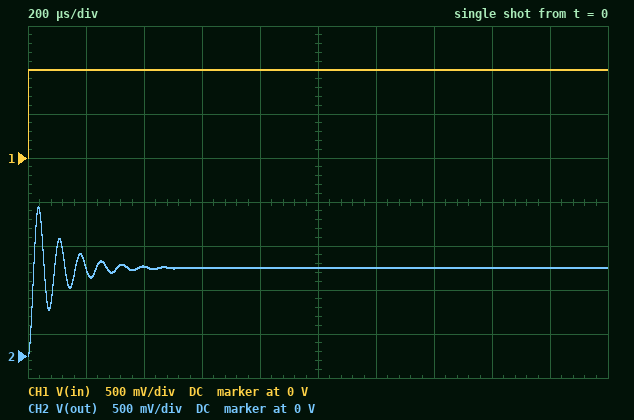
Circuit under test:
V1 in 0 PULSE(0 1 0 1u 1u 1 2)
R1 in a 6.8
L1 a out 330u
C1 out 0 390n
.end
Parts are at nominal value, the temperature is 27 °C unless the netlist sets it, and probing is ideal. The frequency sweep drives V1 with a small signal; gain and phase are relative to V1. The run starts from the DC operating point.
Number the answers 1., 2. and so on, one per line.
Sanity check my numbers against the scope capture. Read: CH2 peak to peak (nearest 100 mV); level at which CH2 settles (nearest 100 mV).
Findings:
1. 1.7 V
2. 1.0 V
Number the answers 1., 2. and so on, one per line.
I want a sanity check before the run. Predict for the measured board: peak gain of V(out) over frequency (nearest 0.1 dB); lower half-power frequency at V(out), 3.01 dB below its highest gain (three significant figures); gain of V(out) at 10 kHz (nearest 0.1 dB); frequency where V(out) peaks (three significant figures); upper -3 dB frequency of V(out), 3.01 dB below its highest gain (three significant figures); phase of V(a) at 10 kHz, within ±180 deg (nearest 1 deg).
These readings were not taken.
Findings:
1. 12.7 dB
2. 12.1 kHz
3. 5.7 dB
4. 13.8 kHz
5. 15.4 kHz
6. -19 deg
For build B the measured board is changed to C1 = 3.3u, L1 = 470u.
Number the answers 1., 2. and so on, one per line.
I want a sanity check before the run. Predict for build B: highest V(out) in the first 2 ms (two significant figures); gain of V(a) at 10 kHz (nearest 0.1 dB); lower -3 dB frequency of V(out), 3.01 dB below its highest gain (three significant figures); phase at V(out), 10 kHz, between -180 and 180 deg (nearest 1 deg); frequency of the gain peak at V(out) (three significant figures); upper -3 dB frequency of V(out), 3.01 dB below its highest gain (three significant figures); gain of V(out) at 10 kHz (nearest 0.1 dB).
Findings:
1. 1.4 V
2. -0.3 dB
3. 2.18 kHz
4. -165 deg
5. 3.70 kHz
6. 4.75 kHz
7. -14.5 dB
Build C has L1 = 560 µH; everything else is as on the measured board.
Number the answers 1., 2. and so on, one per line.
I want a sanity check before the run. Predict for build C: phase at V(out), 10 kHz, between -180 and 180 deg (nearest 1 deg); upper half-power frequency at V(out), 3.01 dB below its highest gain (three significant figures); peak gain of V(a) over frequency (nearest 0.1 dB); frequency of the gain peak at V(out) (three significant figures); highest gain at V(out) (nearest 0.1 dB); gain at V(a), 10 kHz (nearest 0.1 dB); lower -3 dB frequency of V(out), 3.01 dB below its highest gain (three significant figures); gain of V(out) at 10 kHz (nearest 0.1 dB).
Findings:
1. -50 deg
2. 11.6 kHz
3. 0 dB
4. 10.7 kHz
5. 15.0 dB
6. -3.9 dB
7. 9.66 kHz
8. 13.3 dB
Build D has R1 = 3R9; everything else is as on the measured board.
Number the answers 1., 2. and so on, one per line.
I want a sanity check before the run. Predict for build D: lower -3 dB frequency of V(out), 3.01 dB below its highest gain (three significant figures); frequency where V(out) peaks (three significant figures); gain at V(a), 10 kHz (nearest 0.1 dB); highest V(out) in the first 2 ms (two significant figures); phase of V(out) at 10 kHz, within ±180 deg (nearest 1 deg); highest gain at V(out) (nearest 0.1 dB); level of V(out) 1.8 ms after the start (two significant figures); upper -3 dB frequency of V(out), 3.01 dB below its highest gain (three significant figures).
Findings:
1. 13.0 kHz
2. 14.0 kHz
3. -0.2 dB
4. 1.8 V
5. -11 deg
6. 17.5 dB
7. 1.0 V
8. 14.9 kHz
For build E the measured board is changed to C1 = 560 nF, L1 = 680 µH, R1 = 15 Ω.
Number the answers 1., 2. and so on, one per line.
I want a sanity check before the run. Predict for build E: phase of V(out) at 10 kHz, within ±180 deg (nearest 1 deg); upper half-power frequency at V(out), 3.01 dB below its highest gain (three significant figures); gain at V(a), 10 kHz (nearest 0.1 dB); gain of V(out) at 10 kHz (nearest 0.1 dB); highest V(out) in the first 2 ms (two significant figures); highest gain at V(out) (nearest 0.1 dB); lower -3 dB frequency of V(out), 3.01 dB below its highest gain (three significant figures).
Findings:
1. -134 deg
2. 9.40 kHz
3. -3.2 dB
4. 2.7 dB
5. 1.5 V
6. 7.5 dB
7. 5.69 kHz
